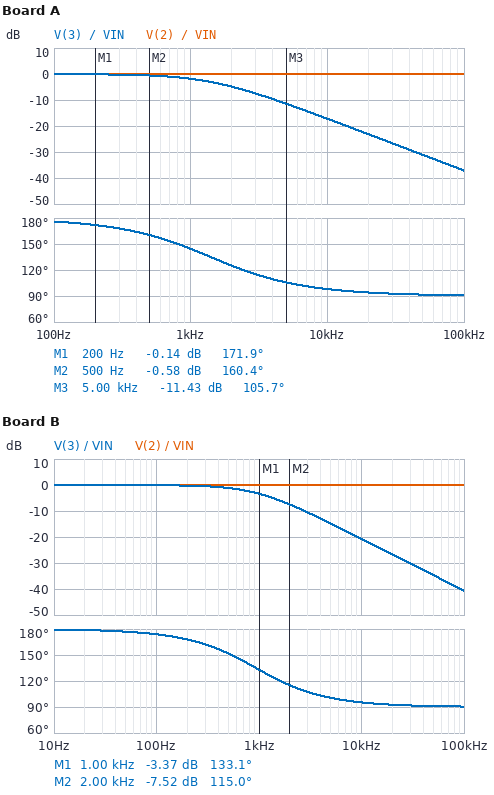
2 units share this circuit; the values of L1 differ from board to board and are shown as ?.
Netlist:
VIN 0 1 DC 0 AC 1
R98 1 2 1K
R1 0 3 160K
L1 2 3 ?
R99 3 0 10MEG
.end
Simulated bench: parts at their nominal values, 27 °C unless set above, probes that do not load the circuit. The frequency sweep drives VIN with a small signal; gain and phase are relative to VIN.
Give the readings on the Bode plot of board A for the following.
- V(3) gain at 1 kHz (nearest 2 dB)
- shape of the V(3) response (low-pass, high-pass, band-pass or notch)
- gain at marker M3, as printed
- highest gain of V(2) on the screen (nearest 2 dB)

-2 dB
low-pass
-11.43 dB
0 dB
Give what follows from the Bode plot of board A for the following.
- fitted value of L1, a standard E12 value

18 H
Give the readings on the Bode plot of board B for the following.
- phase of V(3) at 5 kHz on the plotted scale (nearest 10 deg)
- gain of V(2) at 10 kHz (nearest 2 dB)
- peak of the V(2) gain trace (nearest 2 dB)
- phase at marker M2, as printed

100 deg
0 dB
0 dB
115.0 deg
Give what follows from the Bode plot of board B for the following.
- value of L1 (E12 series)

27 H
